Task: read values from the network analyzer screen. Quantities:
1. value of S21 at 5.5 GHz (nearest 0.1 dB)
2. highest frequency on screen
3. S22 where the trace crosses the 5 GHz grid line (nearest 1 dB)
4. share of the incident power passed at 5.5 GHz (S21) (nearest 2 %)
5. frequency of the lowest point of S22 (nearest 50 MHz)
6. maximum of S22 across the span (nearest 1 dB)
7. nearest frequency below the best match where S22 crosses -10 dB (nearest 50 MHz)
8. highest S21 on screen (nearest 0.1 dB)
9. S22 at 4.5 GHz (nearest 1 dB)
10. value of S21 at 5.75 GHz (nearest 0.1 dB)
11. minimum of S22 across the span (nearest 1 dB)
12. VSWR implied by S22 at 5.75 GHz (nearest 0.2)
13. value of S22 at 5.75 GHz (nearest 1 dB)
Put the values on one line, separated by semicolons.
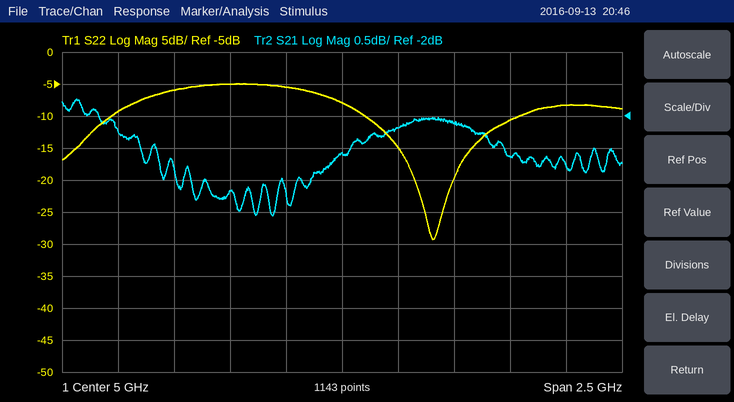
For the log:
-2.1 dB; 6.25 GHz; -8 dB; 62 %; 5.40 GHz; -5 dB; 5.10 GHz; -1.7 dB; -5 dB; -2.6 dB; -29 dB; 1.8; -11 dB
